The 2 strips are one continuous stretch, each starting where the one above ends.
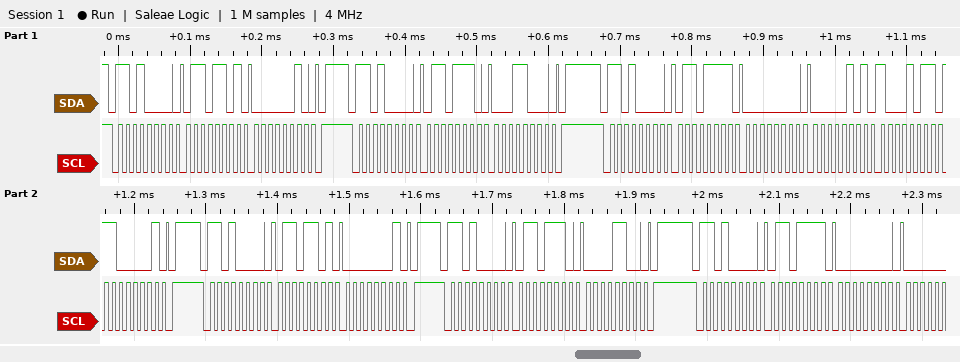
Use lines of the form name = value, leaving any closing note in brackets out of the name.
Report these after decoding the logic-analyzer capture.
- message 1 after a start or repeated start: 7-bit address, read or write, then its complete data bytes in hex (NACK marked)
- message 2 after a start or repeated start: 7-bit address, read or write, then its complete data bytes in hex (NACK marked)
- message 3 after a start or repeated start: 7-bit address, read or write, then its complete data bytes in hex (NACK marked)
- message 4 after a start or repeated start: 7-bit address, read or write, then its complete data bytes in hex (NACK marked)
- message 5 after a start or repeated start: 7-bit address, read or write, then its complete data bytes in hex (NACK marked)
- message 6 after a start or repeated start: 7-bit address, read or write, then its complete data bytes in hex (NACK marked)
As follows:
message 1 after a start or repeated start: 7-bit address, read or write, then its complete data bytes in hex = 0x68 write: 6D 02
message 2 after a start or repeated start: 7-bit address, read or write, then its complete data bytes in hex = 0x68 write: 6E 18
message 3 after a start or repeated start: 7-bit address, read or write, then its complete data bytes in hex = 0x68 write: 6F 00 05 8B C1
message 4 after a start or repeated start: 7-bit address, read or write, then its complete data bytes in hex = 0x68 write: 6D 01
message 5 after a start or repeated start: 7-bit address, read or write, then its complete data bytes in hex = 0x68 write: 6E 0C
message 6 after a start or repeated start: 7-bit address, read or write, then its complete data bytes in hex = 0x68 write: 6F 00
